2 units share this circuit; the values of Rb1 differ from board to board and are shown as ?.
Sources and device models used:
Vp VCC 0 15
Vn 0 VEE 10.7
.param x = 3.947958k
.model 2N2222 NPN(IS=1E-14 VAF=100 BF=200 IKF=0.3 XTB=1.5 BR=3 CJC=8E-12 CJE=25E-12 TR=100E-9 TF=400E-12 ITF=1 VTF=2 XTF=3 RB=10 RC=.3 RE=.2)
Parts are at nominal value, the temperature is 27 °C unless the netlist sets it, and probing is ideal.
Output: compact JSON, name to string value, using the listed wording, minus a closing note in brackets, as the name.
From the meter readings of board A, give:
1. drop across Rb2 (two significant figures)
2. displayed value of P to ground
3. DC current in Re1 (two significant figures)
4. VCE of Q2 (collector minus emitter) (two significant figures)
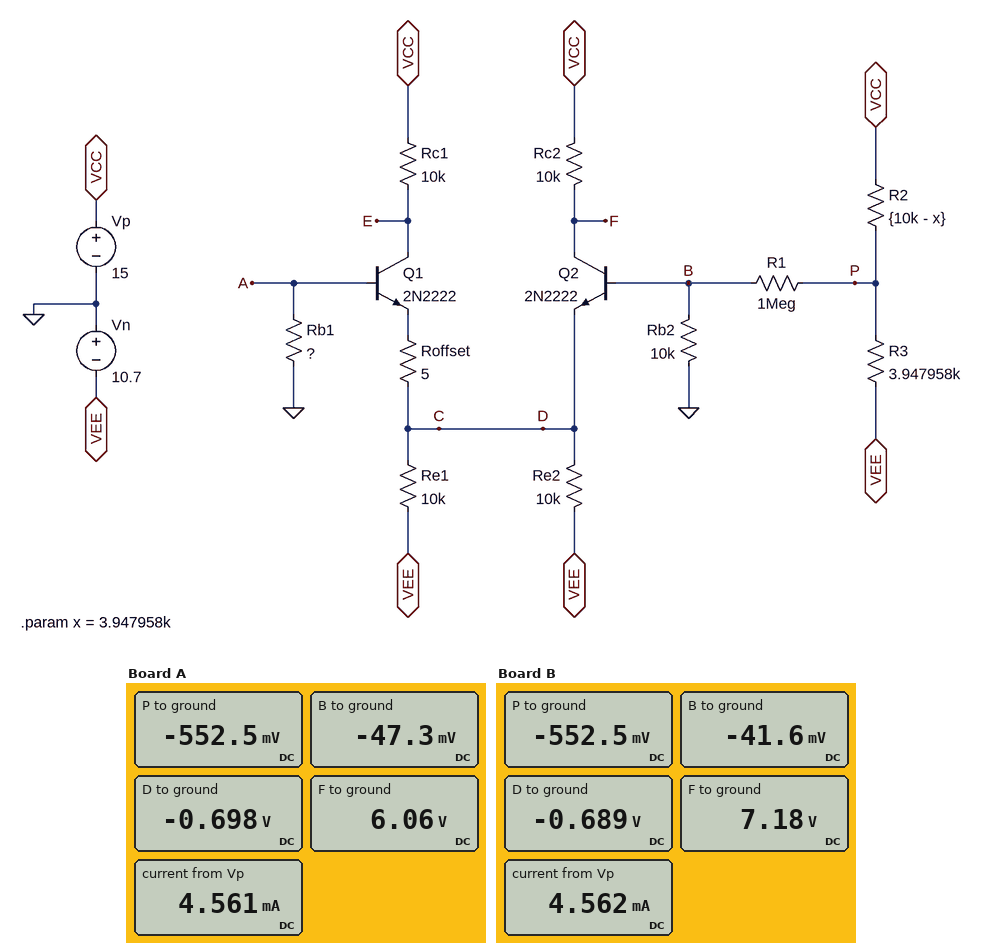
{"drop across Rb2": "47 mV", "displayed value of P to ground": "-552.5 mV", "DC current in Re1": "1.0 mA", "VCE of Q2 (collector minus emitter)": "6.8 V"}
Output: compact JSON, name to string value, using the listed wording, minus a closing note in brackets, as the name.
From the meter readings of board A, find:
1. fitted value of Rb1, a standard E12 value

{"fitted value of Rb1, a standard E12 value": "6.8 kΩ"}
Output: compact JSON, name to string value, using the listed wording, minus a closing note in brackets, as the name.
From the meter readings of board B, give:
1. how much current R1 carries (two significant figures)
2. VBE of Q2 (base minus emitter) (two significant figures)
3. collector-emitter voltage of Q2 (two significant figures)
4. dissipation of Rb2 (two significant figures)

{"how much current R1 carries": "510 nA", "VBE of Q2 (base minus emitter)": "650 mV", "collector-emitter voltage of Q2": "7.9 V", "dissipation of Rb2": "170 nW"}
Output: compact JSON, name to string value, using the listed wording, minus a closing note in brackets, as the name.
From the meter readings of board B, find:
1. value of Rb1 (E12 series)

{"value of Rb1": "3.9 kΩ"}
